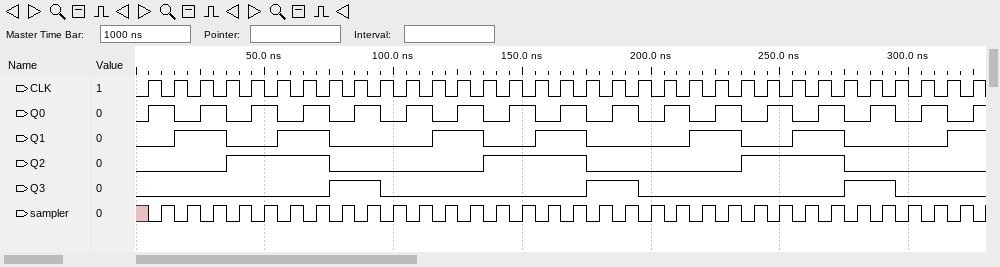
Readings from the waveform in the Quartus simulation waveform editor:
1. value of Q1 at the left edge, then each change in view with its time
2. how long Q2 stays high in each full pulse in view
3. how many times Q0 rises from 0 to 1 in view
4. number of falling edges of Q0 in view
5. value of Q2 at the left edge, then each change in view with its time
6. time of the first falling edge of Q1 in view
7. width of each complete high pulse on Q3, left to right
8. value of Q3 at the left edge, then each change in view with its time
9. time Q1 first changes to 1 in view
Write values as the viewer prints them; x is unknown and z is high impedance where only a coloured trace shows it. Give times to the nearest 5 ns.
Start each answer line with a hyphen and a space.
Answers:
- 0, 1 at 15 ns, 0 at 35 ns, 1 at 55 ns, 0 at 75 ns, 1 at 115 ns, 0 at 135 ns, 1 at 155 ns, 0 at 175 ns, 1 at 215 ns, 0 at 235 ns, 1 at 255 ns, 0 at 275 ns, 1 at 315 ns
- 40 ns, 40 ns, 40 ns
- 17
- 16
- 0, 1 at 35 ns, 0 at 75 ns, 1 at 135 ns, 0 at 175 ns, 1 at 235 ns, 0 at 275 ns
- 35 ns
- 20 ns, 20 ns, 20 ns
- 0, 1 at 75 ns, 0 at 95 ns, 1 at 175 ns, 0 at 195 ns, 1 at 275 ns, 0 at 295 ns
- 15 ns
